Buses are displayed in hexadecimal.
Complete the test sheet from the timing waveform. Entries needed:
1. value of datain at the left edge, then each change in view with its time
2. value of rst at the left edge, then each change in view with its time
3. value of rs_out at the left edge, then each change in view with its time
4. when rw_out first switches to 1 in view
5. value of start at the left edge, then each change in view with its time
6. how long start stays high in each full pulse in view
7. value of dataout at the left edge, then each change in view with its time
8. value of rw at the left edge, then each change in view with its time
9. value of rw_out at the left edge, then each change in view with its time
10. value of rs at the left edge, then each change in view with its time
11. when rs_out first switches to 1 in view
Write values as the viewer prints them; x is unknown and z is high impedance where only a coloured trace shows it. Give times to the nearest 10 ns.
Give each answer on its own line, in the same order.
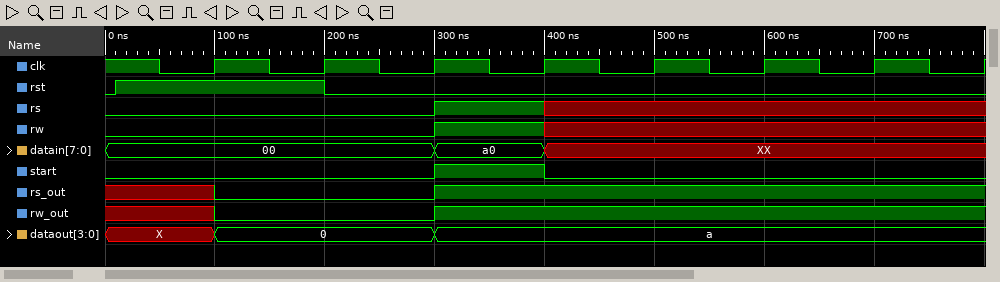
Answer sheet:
00, a0 at 300 ns, XX at 400 ns
0, 1 at 10 ns, 0 at 200 ns
x, 0 at 100 ns, 1 at 300 ns
300 ns
0, 1 at 300 ns, 0 at 400 ns
100 ns
X, 0 at 100 ns, a at 300 ns
0, 1 at 300 ns, x at 400 ns
x, 0 at 100 ns, 1 at 300 ns
0, 1 at 300 ns, x at 400 ns
300 ns
